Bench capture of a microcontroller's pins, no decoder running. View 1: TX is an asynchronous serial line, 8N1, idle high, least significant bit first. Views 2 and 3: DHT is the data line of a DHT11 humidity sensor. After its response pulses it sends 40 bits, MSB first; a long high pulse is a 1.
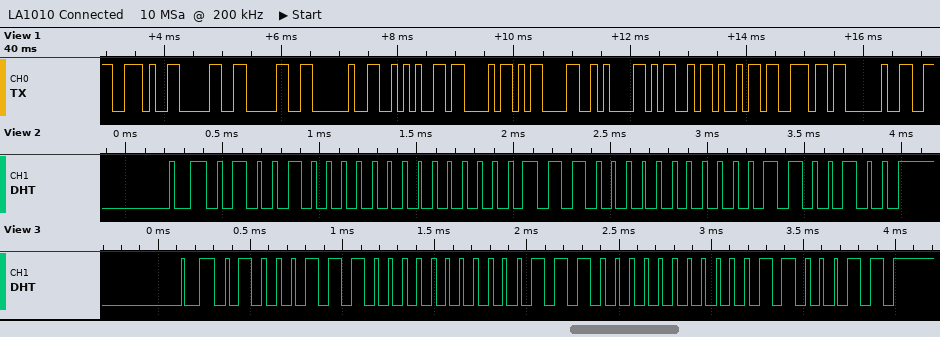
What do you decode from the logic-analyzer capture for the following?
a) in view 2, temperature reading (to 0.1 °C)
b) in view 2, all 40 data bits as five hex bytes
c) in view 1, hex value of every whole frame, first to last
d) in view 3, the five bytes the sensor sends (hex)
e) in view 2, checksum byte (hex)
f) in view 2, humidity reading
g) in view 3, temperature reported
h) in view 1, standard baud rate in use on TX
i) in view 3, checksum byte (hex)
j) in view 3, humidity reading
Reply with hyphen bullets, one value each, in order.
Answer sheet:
- 28.0 °C
- 48 00 1C 00 64
- 2E 30 30 20 2A 43 0D 0A 4D 69 6E 20
- 47 00 1C 00 63
- 0x64
- 72 %
- 28.0 °C
- 9600 baud
- 0x63
- 71 %
